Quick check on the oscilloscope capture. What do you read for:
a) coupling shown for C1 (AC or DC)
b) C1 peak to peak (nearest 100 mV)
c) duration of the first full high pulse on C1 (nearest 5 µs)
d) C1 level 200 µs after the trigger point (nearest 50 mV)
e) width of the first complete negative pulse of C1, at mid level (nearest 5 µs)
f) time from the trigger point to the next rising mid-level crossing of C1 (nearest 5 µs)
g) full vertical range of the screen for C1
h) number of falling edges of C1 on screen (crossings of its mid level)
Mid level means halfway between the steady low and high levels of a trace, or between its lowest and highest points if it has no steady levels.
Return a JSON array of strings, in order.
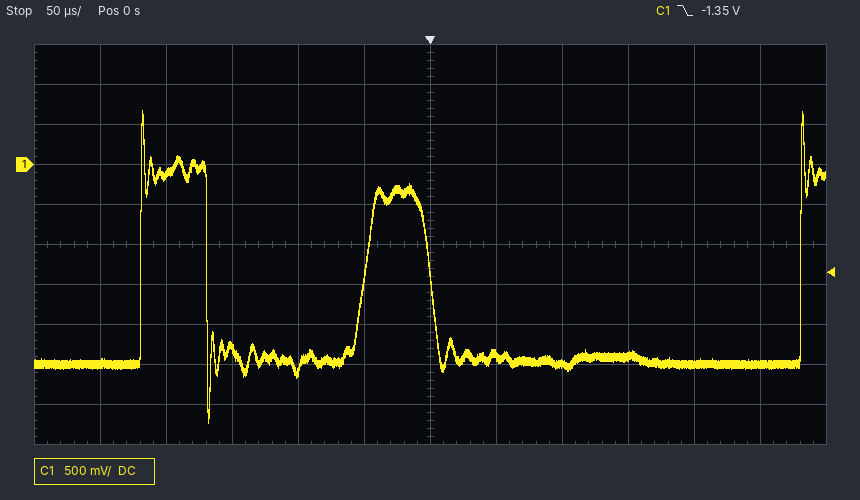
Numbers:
["DC", "3.90 V", "50 µs", "-2.50 V", "120 µs", "280 µs", "5 V", "2"]
